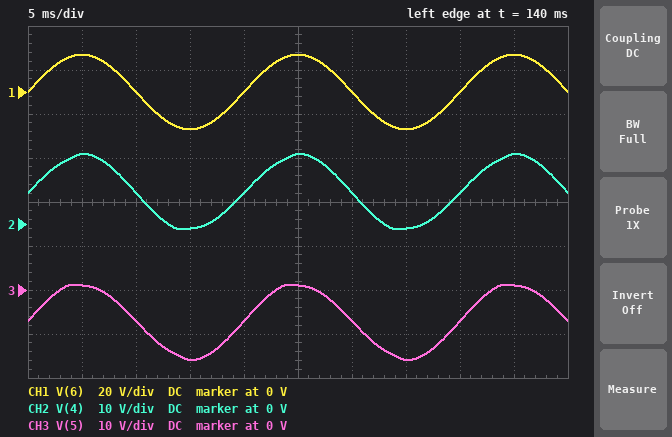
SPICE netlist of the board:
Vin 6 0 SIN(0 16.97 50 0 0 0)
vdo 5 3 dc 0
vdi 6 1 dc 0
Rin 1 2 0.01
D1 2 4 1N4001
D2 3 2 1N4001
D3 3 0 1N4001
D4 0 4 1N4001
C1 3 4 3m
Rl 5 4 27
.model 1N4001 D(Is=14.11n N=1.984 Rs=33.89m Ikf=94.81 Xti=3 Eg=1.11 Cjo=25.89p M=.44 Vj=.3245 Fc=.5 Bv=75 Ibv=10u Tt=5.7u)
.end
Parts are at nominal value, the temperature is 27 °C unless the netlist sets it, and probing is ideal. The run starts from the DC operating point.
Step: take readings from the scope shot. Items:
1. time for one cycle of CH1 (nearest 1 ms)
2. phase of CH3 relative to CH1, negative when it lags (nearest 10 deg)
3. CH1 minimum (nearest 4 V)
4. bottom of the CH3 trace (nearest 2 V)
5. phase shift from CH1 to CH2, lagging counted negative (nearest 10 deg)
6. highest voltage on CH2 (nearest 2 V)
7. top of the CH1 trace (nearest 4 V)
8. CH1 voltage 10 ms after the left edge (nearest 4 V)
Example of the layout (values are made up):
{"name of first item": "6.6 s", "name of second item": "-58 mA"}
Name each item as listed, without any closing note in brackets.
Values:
{"time for one cycle of CH1": "20 ms", "phase of CH3 relative to CH1, negative when it lags": "0 deg", "CH1 minimum": "-16 V", "bottom of the CH3 trace": "-16 V", "phase shift from CH1 to CH2, lagging counted negative": "0 deg", "highest voltage on CH2": "16 V", "top of the CH1 trace": "16 V", "CH1 voltage 10 ms after the left edge": "0 V"}
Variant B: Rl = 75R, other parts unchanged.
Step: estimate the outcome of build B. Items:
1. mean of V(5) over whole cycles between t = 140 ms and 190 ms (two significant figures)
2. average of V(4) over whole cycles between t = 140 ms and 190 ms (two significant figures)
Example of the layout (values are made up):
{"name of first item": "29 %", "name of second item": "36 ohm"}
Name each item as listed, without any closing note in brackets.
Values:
{"mean of V(5) over whole cycles between t = 140 ms and 190 ms": "-7.4 V", "average of V(4) over whole cycles between t = 140 ms and 190 ms": "7.4 V"}
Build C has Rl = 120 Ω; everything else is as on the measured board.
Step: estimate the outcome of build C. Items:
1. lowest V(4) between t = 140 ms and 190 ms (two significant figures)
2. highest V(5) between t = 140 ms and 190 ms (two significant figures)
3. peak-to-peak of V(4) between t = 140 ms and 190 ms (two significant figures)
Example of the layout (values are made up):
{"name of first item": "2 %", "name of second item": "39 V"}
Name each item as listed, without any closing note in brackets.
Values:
{"lowest V(4) between t = 140 ms and 190 ms": "-1.0 V", "highest V(5) between t = 140 ms and 190 ms": "1.0 V", "peak-to-peak of V(4) between t = 140 ms and 190 ms": "17 V"}
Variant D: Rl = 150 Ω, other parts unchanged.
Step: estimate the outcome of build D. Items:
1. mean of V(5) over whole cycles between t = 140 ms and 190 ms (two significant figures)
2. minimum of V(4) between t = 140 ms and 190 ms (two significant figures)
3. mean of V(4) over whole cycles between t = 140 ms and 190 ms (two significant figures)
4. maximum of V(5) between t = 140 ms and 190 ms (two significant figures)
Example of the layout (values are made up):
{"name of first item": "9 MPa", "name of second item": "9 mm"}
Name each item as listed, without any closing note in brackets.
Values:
{"mean of V(5) over whole cycles between t = 140 ms and 190 ms": "-7.5 V", "minimum of V(4) between t = 140 ms and 190 ms": "-990 mV", "mean of V(4) over whole cycles between t = 140 ms and 190 ms": "7.5 V", "maximum of V(5) between t = 140 ms and 190 ms": "990 mV"}
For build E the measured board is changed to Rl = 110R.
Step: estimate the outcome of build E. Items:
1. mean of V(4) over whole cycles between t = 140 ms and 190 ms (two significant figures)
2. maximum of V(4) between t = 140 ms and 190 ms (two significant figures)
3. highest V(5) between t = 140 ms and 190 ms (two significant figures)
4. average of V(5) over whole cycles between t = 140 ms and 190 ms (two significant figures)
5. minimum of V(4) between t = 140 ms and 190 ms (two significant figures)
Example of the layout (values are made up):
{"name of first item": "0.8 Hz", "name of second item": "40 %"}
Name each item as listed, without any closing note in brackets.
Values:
{"mean of V(4) over whole cycles between t = 140 ms and 190 ms": "7.4 V", "maximum of V(4) between t = 140 ms and 190 ms": "16 V", "highest V(5) between t = 140 ms and 190 ms": "1.0 V", "average of V(5) over whole cycles between t = 140 ms and 190 ms": "-7.4 V", "minimum of V(4) between t = 140 ms and 190 ms": "-1.0 V"}
